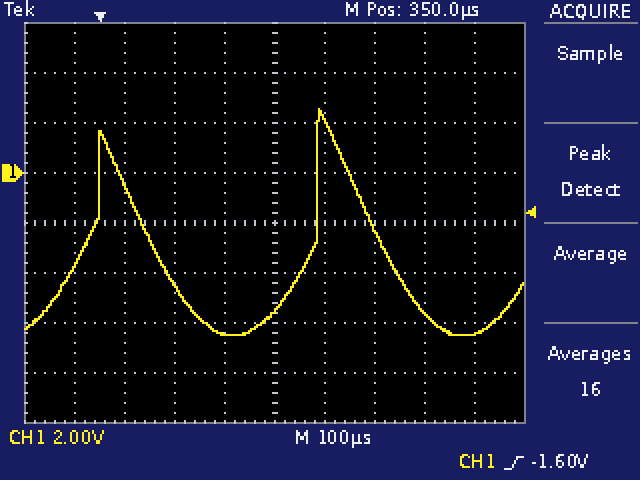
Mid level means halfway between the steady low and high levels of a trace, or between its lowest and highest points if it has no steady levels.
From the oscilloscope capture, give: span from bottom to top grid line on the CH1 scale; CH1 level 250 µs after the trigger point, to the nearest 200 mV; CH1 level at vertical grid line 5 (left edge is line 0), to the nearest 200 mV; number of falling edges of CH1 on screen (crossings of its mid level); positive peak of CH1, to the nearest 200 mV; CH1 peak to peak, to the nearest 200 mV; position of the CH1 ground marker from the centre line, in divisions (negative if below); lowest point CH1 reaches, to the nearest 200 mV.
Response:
16 V
-6.4 V
-5.6 V
2
2.6 V
9.0 V
+1.0 div
-6.4 V
